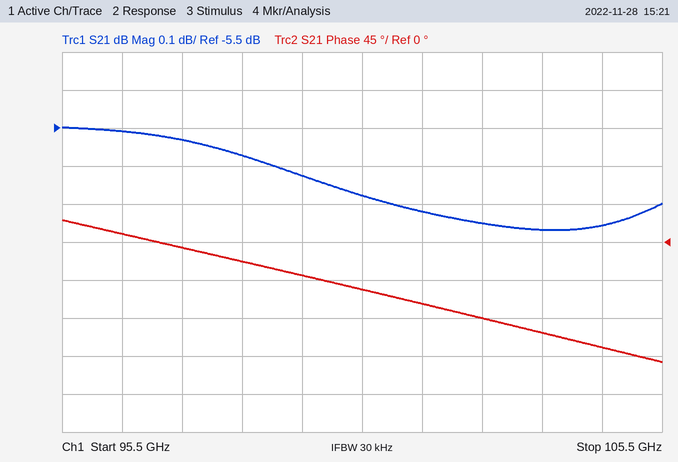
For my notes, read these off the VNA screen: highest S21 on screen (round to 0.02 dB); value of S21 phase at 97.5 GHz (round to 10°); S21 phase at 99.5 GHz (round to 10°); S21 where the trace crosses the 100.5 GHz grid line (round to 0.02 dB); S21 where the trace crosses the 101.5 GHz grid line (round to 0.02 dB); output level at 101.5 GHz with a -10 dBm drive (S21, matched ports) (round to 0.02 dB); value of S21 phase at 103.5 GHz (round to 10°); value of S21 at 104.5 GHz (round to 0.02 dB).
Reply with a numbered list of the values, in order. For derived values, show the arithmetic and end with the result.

1. -5.50 dB
2. -10°
3. -40°
4. -5.68 dB
5. -5.72 dB
6. -10 dBm + (-5.72 dB) = -15.72 dBm
7. -110°
8. -5.76 dB
